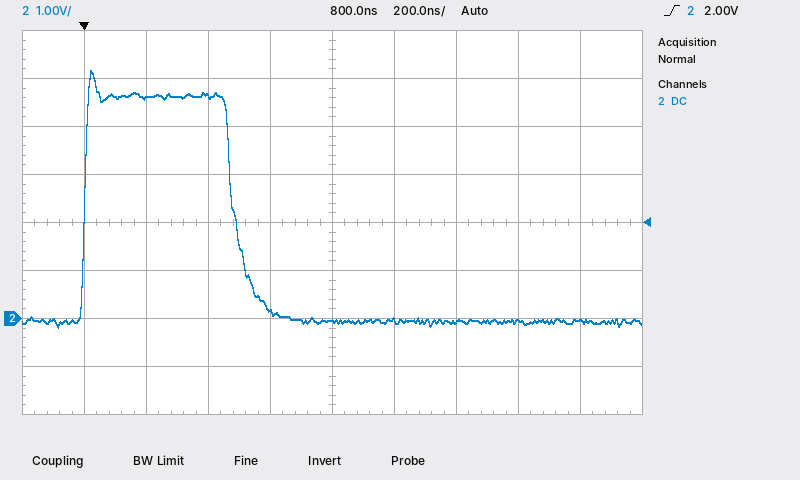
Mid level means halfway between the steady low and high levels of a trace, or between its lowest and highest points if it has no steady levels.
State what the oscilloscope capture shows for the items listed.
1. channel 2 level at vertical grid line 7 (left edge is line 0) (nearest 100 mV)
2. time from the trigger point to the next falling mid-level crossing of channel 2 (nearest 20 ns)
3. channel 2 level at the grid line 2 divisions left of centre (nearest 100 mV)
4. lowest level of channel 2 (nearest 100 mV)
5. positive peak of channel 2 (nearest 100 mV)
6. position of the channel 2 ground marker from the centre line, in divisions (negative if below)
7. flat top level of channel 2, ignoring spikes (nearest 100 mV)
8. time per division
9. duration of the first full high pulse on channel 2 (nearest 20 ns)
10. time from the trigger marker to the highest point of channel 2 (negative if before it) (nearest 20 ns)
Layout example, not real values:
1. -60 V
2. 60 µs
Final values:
1. -100 mV
2. 480 ns
3. 4.6 V
4. -200 mV
5. 5.2 V
6. -2.0 div
7. 4.6 V
8. 200 ns
9. 480 ns
10. +20 ns
